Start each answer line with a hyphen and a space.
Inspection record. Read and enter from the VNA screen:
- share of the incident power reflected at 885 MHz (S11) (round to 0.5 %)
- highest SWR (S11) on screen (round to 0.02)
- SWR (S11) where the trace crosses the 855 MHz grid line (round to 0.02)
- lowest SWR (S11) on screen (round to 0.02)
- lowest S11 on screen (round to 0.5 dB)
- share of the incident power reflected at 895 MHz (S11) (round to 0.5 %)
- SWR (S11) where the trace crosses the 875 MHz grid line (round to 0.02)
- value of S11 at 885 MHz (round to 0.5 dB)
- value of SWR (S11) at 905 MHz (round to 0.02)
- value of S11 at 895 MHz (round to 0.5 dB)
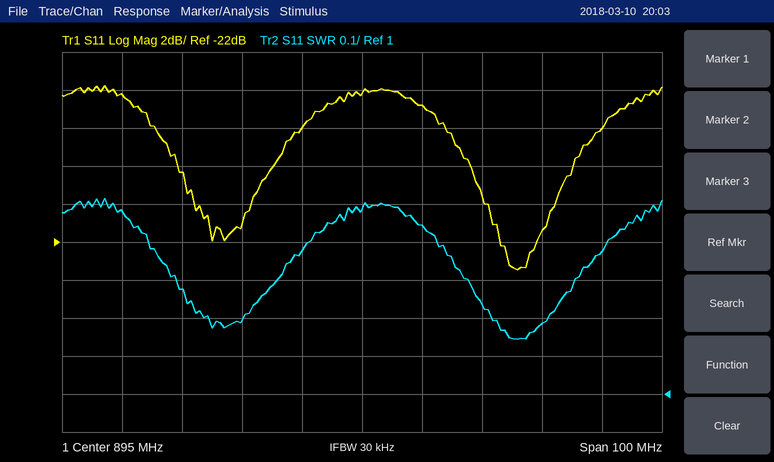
- 2.5 %
- 1.52
- 1.48
- 1.14
- -23.5 dB
- 4.0 %
- 1.20
- -16.0 dB
- 1.44
- -14.0 dB
